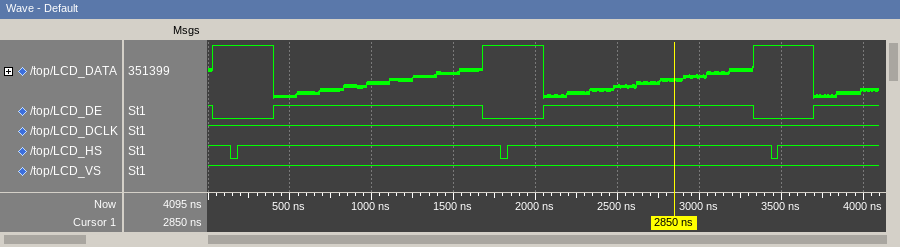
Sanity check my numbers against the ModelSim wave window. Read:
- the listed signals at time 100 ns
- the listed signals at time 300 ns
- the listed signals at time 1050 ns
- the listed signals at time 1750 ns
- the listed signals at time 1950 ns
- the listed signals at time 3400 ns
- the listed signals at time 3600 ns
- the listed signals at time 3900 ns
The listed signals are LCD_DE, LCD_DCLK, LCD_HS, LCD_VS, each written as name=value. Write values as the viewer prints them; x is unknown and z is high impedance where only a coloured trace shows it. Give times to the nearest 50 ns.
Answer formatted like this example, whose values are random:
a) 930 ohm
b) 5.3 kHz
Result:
a) LCD_DE=0, LCD_DCLK=1, LCD_HS=1, LCD_VS=1
b) LCD_DE=0, LCD_DCLK=1, LCD_HS=1, LCD_VS=1
c) LCD_DE=1, LCD_DCLK=1, LCD_HS=1, LCD_VS=1
d) LCD_DE=0, LCD_DCLK=1, LCD_HS=1, LCD_VS=1
e) LCD_DE=0, LCD_DCLK=1, LCD_HS=1, LCD_VS=1
f) LCD_DE=0, LCD_DCLK=1, LCD_HS=1, LCD_VS=1
g) LCD_DE=0, LCD_DCLK=1, LCD_HS=1, LCD_VS=1
h) LCD_DE=1, LCD_DCLK=1, LCD_HS=1, LCD_VS=1
